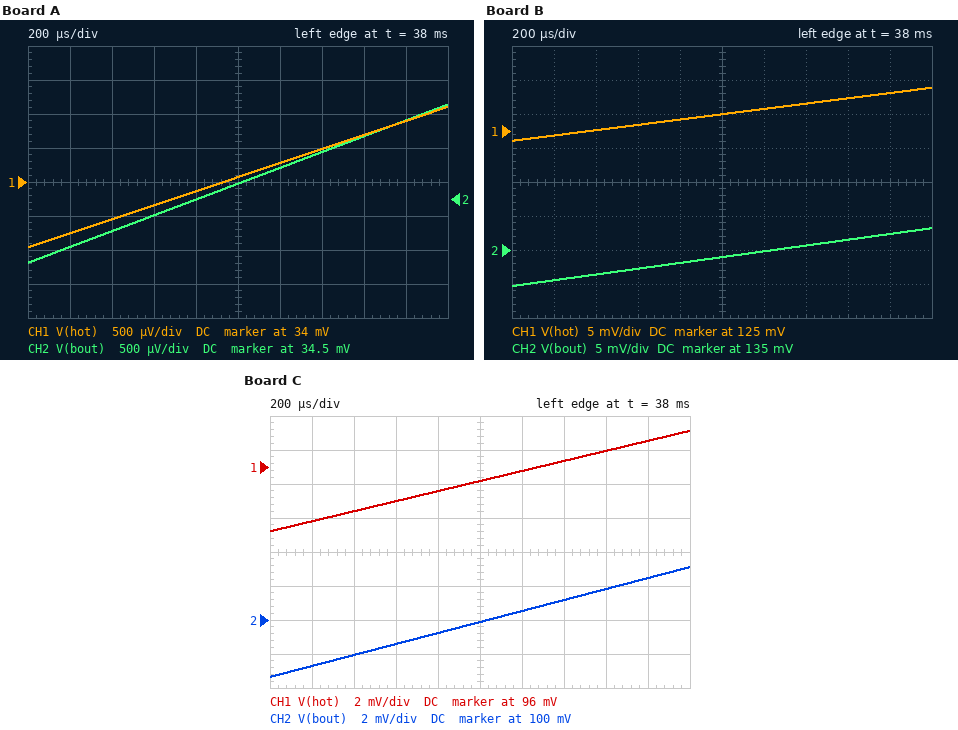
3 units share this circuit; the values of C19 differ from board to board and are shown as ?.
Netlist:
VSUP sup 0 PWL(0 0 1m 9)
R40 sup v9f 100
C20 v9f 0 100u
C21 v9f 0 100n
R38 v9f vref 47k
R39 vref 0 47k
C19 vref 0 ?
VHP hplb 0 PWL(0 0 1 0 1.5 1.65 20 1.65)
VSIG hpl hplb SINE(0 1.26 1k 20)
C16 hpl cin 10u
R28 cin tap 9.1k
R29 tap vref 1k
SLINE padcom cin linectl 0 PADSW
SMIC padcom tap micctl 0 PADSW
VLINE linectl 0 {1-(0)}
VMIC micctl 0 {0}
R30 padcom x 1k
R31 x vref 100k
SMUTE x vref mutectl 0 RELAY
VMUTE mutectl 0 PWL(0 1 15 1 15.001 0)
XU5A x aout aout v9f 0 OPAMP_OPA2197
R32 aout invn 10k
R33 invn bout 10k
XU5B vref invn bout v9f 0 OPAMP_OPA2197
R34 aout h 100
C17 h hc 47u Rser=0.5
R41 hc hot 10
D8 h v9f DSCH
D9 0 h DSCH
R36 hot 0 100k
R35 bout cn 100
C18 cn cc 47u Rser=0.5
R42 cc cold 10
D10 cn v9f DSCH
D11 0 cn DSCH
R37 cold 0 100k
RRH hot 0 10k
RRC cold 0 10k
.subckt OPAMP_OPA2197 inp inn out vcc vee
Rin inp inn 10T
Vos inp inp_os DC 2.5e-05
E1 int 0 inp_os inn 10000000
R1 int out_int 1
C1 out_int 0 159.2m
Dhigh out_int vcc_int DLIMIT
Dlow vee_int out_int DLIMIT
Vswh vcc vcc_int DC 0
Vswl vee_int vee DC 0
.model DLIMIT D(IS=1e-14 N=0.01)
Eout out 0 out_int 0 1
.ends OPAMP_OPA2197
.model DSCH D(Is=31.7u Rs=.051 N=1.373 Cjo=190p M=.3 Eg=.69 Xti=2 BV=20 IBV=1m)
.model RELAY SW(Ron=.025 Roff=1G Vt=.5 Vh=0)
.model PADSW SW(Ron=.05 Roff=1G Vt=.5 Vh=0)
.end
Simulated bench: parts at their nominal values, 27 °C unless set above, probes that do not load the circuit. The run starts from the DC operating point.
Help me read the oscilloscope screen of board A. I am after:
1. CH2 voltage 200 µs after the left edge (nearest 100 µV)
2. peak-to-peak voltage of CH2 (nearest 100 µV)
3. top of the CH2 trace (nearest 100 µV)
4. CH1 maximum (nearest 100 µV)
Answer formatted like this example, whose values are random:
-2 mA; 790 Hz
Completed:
33.8 mV; 2.3 mV; 35.9 mV; 35.1 mV
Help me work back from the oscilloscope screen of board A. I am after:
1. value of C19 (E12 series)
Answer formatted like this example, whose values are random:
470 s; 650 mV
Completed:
150 µF
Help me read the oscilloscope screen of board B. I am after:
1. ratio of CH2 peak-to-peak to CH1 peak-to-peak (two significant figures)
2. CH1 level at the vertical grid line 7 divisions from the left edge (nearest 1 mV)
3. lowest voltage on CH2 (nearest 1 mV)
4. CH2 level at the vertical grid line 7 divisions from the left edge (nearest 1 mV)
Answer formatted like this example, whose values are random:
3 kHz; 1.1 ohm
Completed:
1.1; 129 mV; 130 mV; 136 mV
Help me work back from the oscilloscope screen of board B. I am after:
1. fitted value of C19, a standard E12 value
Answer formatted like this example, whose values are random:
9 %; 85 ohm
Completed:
33 µF
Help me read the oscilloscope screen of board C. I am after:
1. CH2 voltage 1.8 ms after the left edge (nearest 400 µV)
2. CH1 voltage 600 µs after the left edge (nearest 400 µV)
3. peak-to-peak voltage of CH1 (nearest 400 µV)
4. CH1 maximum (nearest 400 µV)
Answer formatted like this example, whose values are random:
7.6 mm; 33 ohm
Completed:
102.4 mV; 94.0 mV; 6.0 mV; 98.0 mV
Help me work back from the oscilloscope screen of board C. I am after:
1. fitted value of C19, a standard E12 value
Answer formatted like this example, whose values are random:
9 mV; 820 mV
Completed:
47 µF
